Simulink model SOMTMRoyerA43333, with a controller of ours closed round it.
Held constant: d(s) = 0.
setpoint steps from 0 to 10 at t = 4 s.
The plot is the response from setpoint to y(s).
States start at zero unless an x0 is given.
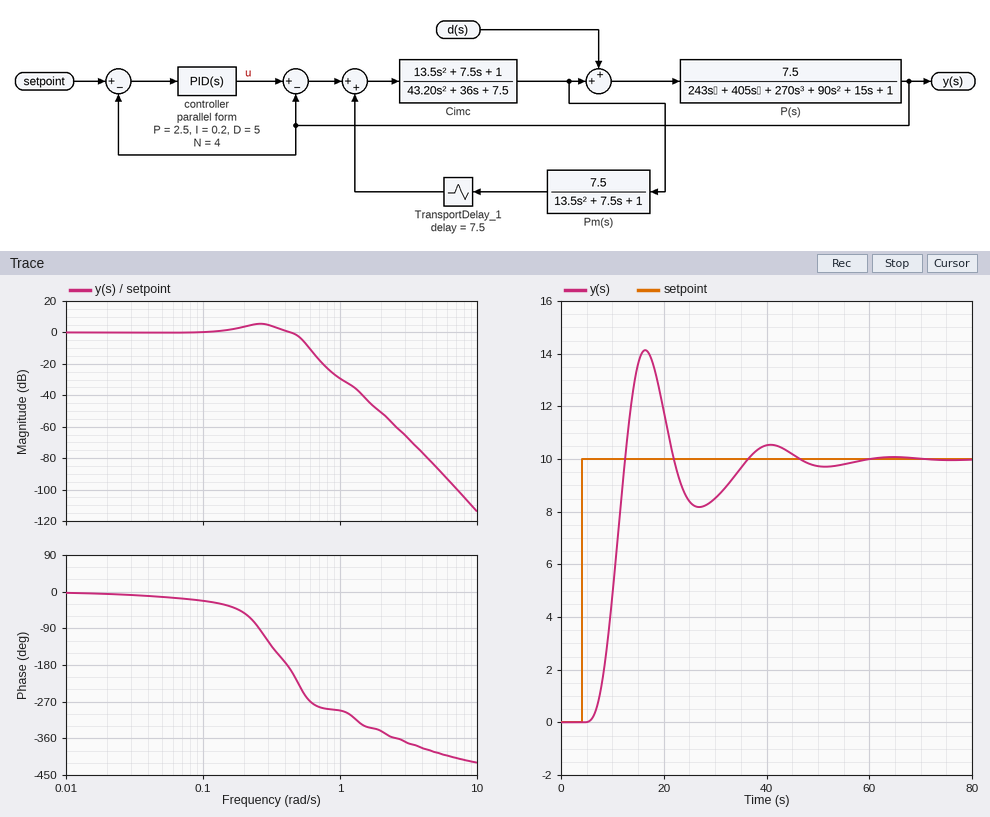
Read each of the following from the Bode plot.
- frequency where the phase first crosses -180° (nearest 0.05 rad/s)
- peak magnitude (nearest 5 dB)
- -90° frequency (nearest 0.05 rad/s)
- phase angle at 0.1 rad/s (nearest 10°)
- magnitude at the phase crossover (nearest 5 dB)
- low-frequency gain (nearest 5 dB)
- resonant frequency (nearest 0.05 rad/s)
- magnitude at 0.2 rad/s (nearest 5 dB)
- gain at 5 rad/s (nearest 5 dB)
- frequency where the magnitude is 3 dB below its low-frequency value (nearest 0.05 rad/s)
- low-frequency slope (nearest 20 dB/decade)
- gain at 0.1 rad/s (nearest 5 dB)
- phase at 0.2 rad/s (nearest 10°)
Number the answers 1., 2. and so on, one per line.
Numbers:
1. 0.40 rad/s
2. 5 dB
3. 0.25 rad/s
4. -20°
5. 0 dB
6. 0 dB
7. 0.25 rad/s
8. 5 dB
9. -85 dB
10. 0.50 rad/s
11. 0 dB/decade
12. 0 dB
13. -50°
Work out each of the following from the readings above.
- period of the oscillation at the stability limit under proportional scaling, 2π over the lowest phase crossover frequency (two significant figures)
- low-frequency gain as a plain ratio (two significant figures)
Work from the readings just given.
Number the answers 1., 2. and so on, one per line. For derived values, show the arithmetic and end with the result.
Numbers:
1. 2π / 0.4 = 16 s
2. 10^(0 / 20) = 1.0
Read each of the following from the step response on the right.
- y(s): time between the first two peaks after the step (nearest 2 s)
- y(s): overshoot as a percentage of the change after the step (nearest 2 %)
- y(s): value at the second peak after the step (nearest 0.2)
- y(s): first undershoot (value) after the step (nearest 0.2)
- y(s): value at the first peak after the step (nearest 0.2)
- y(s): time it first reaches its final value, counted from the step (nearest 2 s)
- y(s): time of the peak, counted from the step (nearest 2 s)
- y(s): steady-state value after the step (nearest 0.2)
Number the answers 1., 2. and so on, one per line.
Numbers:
1. 24 s
2. 42 %
3. 10.6
4. 8.2
5. 14.2
6. 8 s
7. 12 s
8. 10.0
